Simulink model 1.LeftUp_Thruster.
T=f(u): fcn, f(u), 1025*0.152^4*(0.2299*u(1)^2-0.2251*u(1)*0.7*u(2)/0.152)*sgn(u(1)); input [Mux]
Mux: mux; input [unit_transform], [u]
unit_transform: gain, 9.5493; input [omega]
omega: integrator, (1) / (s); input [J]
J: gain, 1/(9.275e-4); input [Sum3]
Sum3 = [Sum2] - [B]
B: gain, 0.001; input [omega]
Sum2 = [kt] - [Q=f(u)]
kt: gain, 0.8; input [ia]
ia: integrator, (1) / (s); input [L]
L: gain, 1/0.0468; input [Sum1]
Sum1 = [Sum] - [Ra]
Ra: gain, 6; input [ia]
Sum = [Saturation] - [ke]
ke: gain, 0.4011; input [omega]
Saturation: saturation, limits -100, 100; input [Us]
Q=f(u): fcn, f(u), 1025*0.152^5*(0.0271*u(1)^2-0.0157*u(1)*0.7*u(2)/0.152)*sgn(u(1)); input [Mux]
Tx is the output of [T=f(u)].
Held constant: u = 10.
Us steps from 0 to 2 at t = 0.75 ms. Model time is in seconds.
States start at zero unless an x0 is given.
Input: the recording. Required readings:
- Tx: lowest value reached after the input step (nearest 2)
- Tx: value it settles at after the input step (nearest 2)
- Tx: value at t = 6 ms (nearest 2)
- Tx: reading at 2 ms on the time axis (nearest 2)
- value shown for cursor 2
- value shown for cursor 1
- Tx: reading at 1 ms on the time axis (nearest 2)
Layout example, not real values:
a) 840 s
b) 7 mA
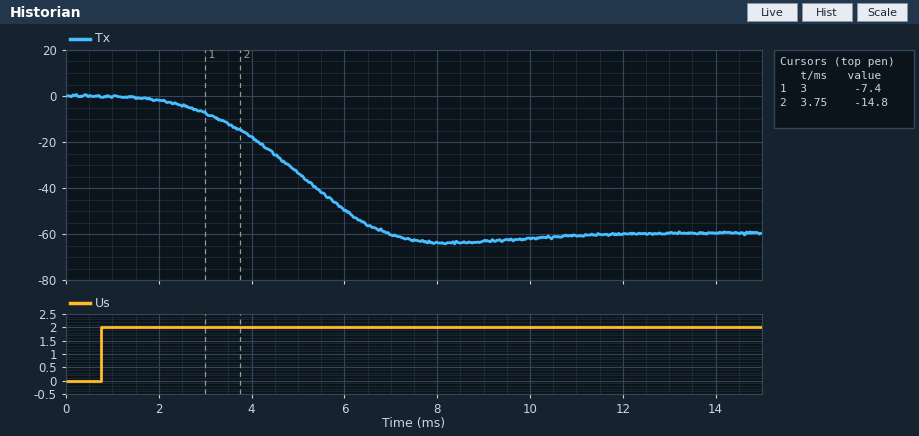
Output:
a) -64
b) -60
c) -50
d) -2
e) -14.8
f) -7.4
g) 0
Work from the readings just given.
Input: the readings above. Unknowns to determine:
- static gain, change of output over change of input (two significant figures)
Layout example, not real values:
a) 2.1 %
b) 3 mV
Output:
a) -30
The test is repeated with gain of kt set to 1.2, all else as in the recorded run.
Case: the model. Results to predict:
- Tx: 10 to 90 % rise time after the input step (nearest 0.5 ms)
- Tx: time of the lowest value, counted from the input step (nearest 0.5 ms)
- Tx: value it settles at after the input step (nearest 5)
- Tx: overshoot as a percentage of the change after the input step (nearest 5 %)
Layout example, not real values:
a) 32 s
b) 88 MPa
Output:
a) 3.0 ms
b) 6.5 ms
c) -60
d) 10 %
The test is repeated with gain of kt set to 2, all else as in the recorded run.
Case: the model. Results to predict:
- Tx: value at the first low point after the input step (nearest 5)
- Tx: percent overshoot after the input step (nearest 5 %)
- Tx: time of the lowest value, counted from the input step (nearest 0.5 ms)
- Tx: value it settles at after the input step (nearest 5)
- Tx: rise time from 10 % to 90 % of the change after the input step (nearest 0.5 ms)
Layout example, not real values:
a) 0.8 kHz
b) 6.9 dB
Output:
a) -65
b) 15 %
c) 5.5 ms
d) -55
e) 2.5 ms
